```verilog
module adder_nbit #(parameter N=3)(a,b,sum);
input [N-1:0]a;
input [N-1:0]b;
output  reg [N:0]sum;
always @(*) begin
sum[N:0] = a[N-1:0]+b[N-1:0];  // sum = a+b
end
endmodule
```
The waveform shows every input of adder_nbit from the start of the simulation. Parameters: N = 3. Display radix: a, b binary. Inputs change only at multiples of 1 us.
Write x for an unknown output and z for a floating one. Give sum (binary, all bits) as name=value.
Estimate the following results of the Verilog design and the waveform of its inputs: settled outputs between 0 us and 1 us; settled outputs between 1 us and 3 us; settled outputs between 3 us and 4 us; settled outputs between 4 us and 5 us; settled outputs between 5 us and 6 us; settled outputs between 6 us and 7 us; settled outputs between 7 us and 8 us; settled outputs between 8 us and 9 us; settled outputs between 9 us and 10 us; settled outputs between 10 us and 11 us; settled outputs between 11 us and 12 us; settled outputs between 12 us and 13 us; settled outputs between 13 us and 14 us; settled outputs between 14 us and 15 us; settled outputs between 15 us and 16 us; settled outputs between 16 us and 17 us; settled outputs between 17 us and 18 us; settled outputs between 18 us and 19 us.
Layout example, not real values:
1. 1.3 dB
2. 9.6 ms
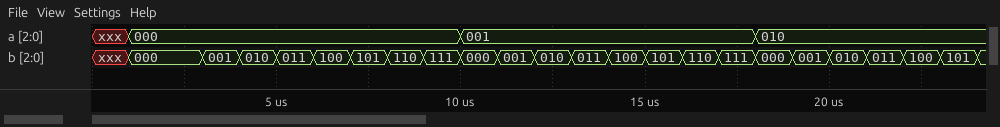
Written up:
1. sum=x
2. sum=0000
3. sum=0001
4. sum=0010
5. sum=0011
6. sum=0100
7. sum=0101
8. sum=0110
9. sum=0111
10. sum=0001
11. sum=0010
12. sum=0011
13. sum=0100
14. sum=0101
15. sum=0110
16. sum=0111
17. sum=1000
18. sum=0010
